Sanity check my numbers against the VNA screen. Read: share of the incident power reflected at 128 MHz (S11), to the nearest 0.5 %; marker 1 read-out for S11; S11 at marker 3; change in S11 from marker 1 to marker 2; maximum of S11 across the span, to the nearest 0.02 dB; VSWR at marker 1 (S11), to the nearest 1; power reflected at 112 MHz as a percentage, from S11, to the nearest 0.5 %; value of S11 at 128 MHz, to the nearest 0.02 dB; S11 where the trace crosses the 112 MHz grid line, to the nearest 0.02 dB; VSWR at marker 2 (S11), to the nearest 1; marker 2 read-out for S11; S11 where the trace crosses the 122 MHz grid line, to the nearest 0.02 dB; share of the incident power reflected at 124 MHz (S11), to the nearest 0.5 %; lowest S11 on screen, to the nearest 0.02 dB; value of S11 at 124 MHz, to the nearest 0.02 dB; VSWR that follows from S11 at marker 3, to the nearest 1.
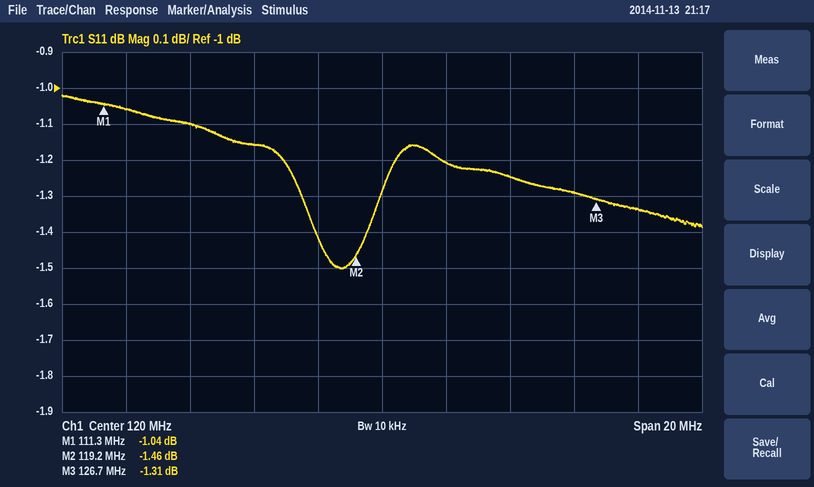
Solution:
73.5 %
-1.04 dB
-1.31 dB
-0.42 dB
-1.02 dB
17
78.5 %
-1.34 dB
-1.06 dB
12
-1.46 dB
-1.20 dB
75.0 %
-1.50 dB
-1.24 dB
13
